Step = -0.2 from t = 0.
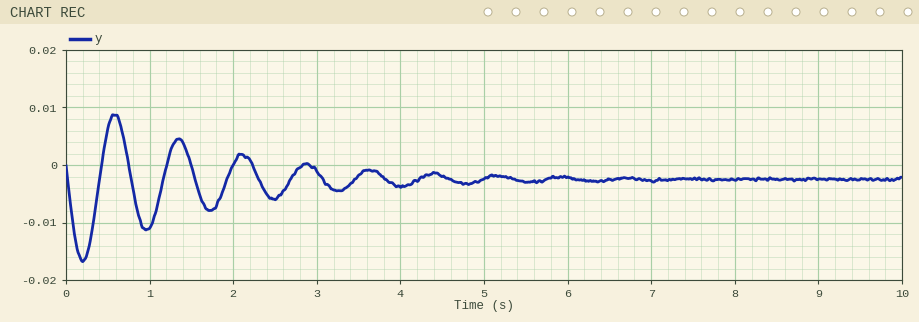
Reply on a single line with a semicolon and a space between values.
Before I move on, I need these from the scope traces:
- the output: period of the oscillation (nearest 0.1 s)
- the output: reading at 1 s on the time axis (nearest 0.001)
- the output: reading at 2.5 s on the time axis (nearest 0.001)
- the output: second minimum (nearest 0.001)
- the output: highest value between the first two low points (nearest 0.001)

0.8 s; -0.011; -0.006; -0.011; 0.009
